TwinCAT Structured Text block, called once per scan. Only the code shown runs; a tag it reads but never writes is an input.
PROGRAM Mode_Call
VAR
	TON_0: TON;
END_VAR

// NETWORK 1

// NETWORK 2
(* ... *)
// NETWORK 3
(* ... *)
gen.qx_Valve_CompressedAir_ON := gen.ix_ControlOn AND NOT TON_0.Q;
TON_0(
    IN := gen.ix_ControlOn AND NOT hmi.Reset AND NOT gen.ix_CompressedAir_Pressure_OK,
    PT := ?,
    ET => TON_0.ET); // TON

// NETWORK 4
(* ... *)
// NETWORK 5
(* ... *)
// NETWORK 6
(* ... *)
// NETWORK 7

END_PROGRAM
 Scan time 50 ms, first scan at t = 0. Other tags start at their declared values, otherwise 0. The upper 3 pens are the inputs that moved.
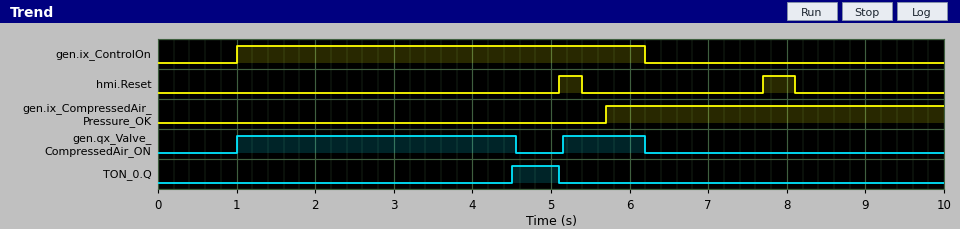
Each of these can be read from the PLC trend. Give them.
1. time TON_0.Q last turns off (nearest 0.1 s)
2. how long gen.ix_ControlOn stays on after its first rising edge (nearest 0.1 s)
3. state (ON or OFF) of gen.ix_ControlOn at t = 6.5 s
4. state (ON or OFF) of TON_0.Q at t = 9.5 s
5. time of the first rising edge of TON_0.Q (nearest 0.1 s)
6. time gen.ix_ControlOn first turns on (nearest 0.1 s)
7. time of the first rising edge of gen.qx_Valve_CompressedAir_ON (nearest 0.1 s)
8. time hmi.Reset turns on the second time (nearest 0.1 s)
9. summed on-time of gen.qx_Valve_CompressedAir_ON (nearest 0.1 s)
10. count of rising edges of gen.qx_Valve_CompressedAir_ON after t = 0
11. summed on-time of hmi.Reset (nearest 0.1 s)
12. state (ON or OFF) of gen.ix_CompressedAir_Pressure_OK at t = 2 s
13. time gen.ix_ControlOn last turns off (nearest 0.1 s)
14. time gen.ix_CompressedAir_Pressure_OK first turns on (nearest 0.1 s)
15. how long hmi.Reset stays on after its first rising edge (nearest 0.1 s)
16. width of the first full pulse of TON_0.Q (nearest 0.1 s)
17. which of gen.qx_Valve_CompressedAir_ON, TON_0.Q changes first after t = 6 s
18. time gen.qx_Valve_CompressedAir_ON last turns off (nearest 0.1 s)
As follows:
5.1 s
5.2 s
OFF
OFF
4.5 s
1.0 s
1.0 s
7.7 s
4.6 s
2
0.7 s
OFF
6.2 s
5.7 s
0.3 s
0.6 s
gen.qx_Valve_CompressedAir_ON
6.2 s
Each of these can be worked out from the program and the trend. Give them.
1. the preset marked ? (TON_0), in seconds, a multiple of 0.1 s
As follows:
3.5 s
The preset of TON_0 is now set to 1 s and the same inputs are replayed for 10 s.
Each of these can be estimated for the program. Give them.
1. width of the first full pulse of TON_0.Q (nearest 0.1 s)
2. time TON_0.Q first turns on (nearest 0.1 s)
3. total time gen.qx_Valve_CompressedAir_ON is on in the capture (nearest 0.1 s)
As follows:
3.1 s
2.0 s
2.1 s
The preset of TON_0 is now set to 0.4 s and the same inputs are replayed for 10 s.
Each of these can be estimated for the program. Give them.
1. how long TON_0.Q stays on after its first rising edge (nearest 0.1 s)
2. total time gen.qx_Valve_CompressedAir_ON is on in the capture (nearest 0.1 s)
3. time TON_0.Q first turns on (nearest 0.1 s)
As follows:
3.7 s
1.5 s
1.4 s
